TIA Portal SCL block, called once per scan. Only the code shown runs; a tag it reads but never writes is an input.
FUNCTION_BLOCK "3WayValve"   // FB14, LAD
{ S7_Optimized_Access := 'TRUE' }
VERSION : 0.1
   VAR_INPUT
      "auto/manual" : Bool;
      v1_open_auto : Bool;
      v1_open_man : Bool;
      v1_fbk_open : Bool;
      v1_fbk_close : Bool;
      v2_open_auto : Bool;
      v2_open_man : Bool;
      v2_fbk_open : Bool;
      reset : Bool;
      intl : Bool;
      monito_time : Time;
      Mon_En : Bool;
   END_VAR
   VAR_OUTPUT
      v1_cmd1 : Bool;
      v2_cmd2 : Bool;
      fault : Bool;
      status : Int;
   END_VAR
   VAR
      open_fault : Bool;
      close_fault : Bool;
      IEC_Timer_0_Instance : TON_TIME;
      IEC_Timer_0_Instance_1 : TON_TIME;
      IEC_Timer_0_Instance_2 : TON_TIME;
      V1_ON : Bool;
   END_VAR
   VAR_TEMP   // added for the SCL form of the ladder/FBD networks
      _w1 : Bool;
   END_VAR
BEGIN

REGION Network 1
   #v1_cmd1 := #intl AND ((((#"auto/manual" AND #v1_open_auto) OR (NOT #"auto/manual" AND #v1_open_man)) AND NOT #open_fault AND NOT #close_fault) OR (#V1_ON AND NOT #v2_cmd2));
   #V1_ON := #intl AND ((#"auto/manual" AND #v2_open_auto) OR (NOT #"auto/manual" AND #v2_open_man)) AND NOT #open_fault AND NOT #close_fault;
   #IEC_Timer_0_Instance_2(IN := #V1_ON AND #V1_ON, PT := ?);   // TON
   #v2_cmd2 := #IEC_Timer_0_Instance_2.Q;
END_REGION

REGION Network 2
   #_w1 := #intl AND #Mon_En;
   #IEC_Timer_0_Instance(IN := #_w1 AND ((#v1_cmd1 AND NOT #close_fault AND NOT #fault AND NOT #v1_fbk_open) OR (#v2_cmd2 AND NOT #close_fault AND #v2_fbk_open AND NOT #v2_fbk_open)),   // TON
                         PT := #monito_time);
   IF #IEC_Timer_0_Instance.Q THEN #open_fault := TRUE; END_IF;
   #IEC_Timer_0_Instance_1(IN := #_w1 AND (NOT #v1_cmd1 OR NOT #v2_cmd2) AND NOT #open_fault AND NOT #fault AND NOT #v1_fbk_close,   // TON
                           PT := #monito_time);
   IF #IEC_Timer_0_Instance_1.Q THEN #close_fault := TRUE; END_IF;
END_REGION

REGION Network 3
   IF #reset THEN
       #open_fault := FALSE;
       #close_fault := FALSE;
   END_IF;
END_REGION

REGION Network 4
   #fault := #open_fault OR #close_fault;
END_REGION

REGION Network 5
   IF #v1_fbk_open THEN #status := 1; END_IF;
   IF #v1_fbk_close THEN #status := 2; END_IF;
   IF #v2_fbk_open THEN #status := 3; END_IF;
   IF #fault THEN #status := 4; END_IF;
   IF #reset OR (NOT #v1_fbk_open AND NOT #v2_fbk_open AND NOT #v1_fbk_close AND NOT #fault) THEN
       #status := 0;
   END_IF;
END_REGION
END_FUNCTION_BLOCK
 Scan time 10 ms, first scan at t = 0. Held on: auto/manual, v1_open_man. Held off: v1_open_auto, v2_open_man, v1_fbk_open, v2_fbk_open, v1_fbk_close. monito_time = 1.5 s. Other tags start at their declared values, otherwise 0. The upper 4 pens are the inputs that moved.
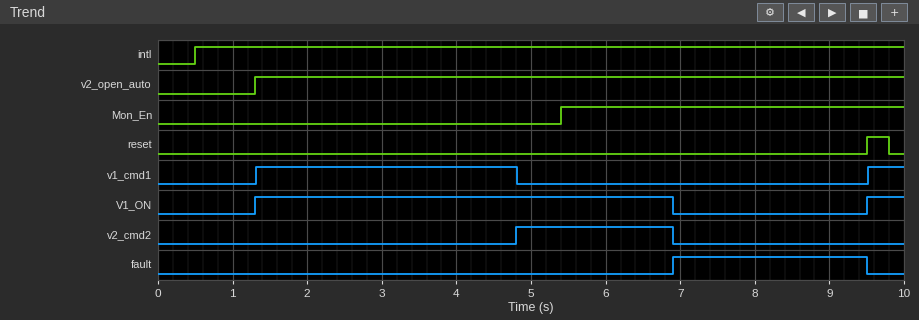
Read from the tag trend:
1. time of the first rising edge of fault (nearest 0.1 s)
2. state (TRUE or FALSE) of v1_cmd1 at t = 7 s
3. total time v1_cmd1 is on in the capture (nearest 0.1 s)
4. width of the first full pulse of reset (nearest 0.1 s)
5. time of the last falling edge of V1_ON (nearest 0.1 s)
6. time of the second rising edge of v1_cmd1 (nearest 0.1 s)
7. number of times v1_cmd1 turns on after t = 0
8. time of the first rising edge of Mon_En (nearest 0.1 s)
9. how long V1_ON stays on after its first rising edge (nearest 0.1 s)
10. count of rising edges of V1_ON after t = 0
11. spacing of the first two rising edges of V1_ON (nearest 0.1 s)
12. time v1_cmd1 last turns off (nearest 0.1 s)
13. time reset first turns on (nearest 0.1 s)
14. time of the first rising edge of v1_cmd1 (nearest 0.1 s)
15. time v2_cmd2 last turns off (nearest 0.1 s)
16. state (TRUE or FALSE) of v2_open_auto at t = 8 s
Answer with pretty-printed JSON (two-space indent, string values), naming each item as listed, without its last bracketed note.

{
  "time of the first rising edge of fault": "6.9 s",
  "state (TRUE or FALSE) of v1_cmd1 at t = 7 s": "FALSE",
  "total time v1_cmd1 is on in the capture": "4.0 s",
  "width of the first full pulse of reset": "0.3 s",
  "time of the last falling edge of V1_ON": "6.9 s",
  "time of the second rising edge of v1_cmd1": "9.5 s",
  "number of times v1_cmd1 turns on after t = 0": "2",
  "time of the first rising edge of Mon_En": "5.4 s",
  "how long V1_ON stays on after its first rising edge": "5.6 s",
  "count of rising edges of V1_ON after t = 0": "2",
  "spacing of the first two rising edges of V1_ON": "8.2 s",
  "time v1_cmd1 last turns off": "4.8 s",
  "time reset first turns on": "9.5 s",
  "time of the first rising edge of v1_cmd1": "1.3 s",
  "time v2_cmd2 last turns off": "6.9 s",
  "state (TRUE or FALSE) of v2_open_auto at t = 8 s": "TRUE"
}
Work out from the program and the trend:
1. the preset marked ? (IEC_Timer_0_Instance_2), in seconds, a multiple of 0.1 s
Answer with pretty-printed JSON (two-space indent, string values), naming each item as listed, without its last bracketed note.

{
  "the preset marked ? (IEC_Timer_0_Instance_2), in seconds, a multiple of 0.1 s": "3.5 s"
}
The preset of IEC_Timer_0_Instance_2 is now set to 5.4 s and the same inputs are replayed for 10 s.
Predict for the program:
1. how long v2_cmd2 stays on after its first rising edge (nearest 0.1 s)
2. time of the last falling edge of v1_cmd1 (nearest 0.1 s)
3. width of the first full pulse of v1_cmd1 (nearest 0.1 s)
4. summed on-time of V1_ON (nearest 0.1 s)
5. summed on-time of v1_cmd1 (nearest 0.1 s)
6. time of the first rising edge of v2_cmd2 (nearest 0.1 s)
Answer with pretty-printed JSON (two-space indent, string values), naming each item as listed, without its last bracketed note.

{
  "how long v2_cmd2 stays on after its first rising edge": "1.5 s",
  "time of the last falling edge of v1_cmd1": "6.7 s",
  "width of the first full pulse of v1_cmd1": "5.4 s",
  "summed on-time of V1_ON": "7.4 s",
  "summed on-time of v1_cmd1": "5.9 s",
  "time of the first rising edge of v2_cmd2": "6.7 s"
}
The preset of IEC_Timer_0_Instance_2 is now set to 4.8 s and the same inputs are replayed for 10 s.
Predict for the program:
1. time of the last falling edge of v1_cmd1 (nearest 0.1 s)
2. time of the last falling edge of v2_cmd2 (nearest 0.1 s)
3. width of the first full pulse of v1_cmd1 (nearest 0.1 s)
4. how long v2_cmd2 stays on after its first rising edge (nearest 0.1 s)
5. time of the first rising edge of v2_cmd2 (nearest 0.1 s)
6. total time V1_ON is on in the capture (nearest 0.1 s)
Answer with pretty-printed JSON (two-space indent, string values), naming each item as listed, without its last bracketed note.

{
  "time of the last falling edge of v1_cmd1": "6.1 s",
  "time of the last falling edge of v2_cmd2": "7.6 s",
  "width of the first full pulse of v1_cmd1": "4.8 s",
  "how long v2_cmd2 stays on after its first rising edge": "1.5 s",
  "time of the first rising edge of v2_cmd2": "6.1 s",
  "total time V1_ON is on in the capture": "6.8 s"
}
